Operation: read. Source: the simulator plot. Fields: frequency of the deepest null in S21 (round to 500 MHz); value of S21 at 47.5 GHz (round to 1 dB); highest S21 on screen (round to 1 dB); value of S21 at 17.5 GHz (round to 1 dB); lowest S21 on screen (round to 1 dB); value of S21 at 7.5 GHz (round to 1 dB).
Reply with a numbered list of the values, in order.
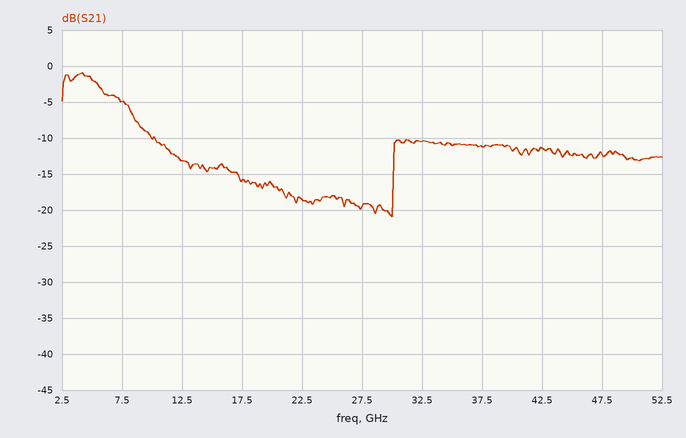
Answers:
1. 30.0 GHz
2. -12 dB
3. -1 dB
4. -16 dB
5. -21 dB
6. -5 dB
